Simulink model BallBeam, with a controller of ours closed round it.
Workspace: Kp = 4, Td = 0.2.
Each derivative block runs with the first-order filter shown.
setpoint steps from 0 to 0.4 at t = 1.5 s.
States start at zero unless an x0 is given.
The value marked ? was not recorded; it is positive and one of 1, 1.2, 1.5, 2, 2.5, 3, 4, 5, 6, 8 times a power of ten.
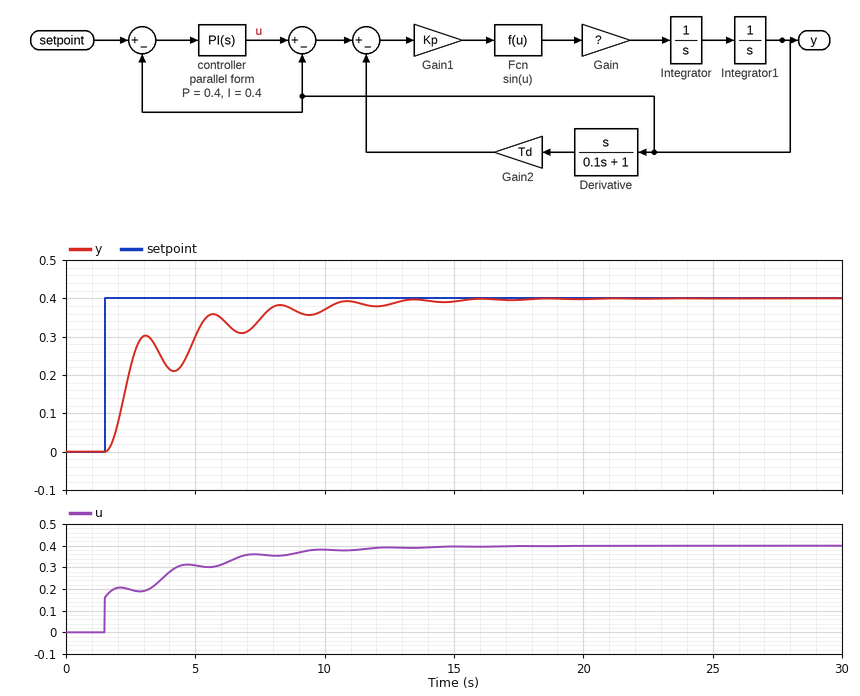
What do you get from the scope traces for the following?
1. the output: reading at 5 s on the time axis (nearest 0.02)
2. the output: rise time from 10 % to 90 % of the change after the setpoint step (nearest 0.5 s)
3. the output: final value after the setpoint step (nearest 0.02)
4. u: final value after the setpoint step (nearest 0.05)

0.30
6.0 s
0.40
0.40
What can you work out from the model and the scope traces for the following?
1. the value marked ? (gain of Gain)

1
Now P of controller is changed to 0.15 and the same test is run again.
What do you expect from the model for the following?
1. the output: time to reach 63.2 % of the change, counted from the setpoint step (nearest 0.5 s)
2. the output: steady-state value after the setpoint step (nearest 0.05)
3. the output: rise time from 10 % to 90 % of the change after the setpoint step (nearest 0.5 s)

1.5 s
0.40
4.0 s
